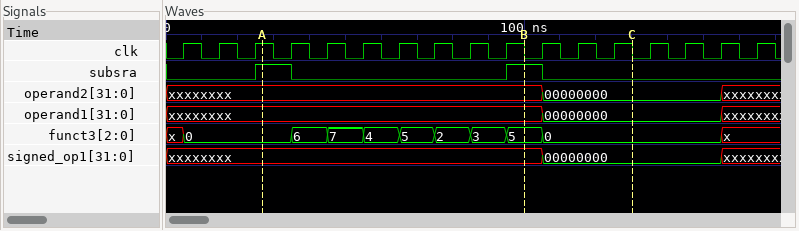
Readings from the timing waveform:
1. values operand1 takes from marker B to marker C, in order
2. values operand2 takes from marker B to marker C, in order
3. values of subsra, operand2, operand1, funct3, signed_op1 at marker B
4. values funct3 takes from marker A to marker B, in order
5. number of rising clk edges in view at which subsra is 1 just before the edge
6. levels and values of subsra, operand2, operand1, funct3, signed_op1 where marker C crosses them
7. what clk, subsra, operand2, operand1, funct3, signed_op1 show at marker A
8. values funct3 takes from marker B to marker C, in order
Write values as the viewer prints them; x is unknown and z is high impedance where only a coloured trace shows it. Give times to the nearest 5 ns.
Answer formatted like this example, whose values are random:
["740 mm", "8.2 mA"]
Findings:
["xxxxxxxx, 00000000", "xxxxxxxx, 00000000", "subsra=1, operand2=xxxxxxxx, operand1=xxxxxxxx, funct3=5, signed_op1=xxxxxxxx", "0, 6, 7, 4, 5, 2, 3, 5", "2", "subsra=0, operand2=00000000, operand1=00000000, funct3=0, signed_op1=00000000", "clk=1, subsra=1, operand2=xxxxxxxx, operand1=xxxxxxxx, funct3=0, signed_op1=xxxxxxxx", "5, 0"]
